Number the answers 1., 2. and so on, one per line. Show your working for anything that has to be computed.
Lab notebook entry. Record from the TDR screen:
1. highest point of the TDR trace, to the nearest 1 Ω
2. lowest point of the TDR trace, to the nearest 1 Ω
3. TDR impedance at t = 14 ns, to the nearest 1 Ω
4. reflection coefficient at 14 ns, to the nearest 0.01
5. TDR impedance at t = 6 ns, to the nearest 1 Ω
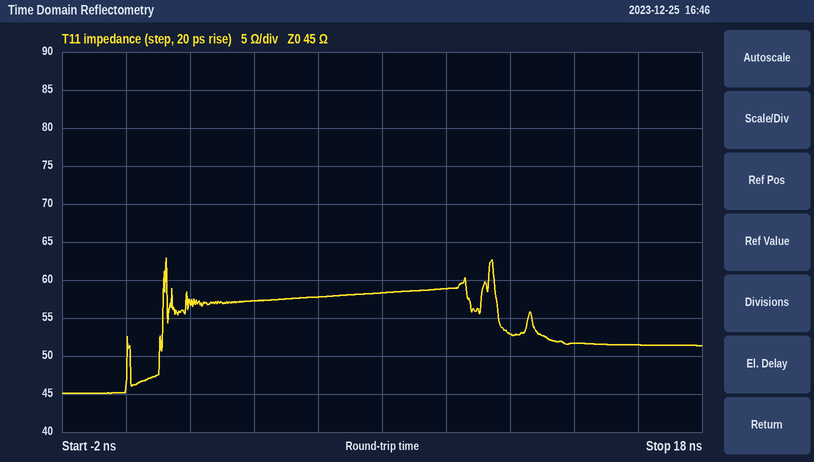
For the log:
1. 63 Ω
2. 45 Ω
3. 52 Ω
4. (52 − 45)/(52 + 45) ≈ +0.07
5. 58 Ω
